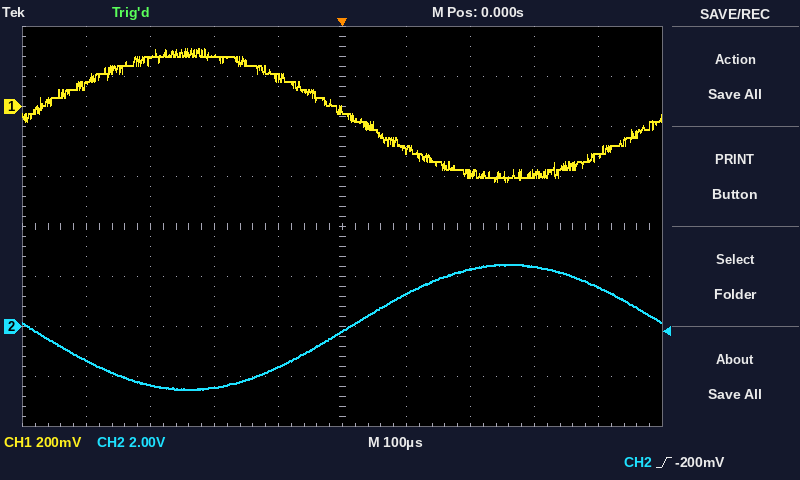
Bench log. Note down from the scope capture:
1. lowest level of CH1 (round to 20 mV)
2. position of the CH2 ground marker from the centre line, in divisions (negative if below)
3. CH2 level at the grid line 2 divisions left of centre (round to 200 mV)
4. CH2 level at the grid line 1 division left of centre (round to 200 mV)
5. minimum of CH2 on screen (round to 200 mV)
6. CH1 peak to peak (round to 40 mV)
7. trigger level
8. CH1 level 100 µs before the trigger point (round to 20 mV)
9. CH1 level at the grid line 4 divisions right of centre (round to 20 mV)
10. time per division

-300 mV
-2.0 div
-2.4 V
-1.6 V
-2.6 V
520 mV
-200 mV
120 mV
-200 mV
100 µs
